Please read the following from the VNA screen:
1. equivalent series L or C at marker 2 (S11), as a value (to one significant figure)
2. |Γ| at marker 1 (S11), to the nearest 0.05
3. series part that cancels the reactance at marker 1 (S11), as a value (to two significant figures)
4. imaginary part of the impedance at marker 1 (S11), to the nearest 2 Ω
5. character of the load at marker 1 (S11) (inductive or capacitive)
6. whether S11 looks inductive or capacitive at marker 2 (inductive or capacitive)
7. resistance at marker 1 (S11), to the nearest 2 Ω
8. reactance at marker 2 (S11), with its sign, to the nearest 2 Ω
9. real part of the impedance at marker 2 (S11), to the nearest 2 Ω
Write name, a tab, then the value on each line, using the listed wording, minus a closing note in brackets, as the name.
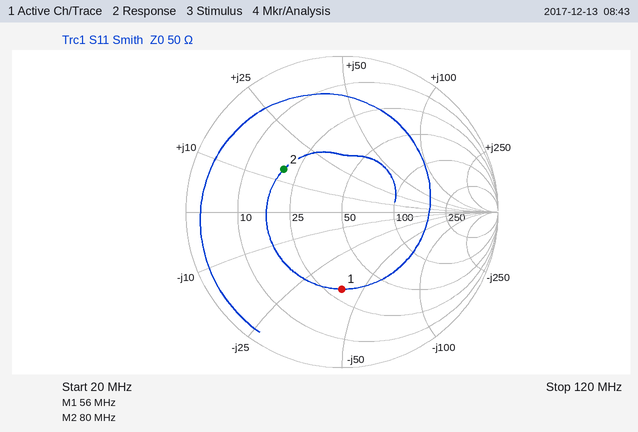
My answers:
equivalent series L or C at marker 2 (S11), as a value	30 nH
|Γ| at marker 1 (S11), to the nearest 0.05	0.50
series part that cancels the reactance at marker 1 (S11), as a value	110 nH
imaginary part of the impedance at marker 1 (S11), to the nearest 2 Ω	-40 Ω
character of the load at marker 1 (S11)	capacitive
whether S11 looks inductive or capacitive at marker 2	inductive
resistance at marker 1 (S11), to the nearest 2 Ω	30 Ω
reactance at marker 2 (S11), with its sign, to the nearest 2 Ω	+14 Ω
real part of the impedance at marker 2 (S11), to the nearest 2 Ω	20 Ω
